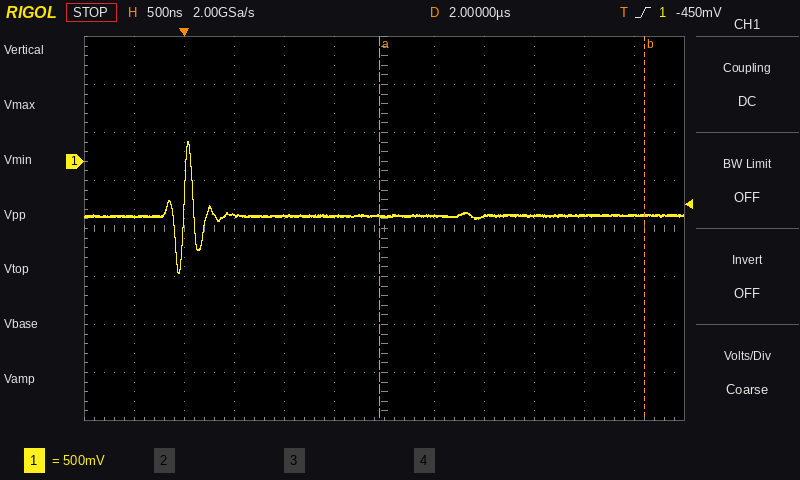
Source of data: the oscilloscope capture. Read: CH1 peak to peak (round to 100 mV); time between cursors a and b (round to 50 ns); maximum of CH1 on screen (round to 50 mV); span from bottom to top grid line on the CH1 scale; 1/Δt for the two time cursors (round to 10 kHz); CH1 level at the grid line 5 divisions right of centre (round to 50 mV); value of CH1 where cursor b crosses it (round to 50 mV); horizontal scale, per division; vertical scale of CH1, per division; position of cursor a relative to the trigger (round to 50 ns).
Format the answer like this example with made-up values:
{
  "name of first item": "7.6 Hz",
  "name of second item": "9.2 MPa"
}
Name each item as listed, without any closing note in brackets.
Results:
{
  "CH1 peak to peak": "1.40 V",
  "time between cursors a and b": "2.65 µs",
  "maximum of CH1 on screen": "200 mV",
  "span from bottom to top grid line on the CH1 scale": "4 V",
  "1/Δt for the two time cursors": "380 kHz",
  "CH1 level at the grid line 5 divisions right of centre": "-550 mV",
  "value of CH1 where cursor b crosses it": "-550 mV",
  "horizontal scale, per division": "500 ns",
  "vertical scale of CH1, per division": "500 mV",
  "position of cursor a relative to the trigger": "+1.95 µs"
}
